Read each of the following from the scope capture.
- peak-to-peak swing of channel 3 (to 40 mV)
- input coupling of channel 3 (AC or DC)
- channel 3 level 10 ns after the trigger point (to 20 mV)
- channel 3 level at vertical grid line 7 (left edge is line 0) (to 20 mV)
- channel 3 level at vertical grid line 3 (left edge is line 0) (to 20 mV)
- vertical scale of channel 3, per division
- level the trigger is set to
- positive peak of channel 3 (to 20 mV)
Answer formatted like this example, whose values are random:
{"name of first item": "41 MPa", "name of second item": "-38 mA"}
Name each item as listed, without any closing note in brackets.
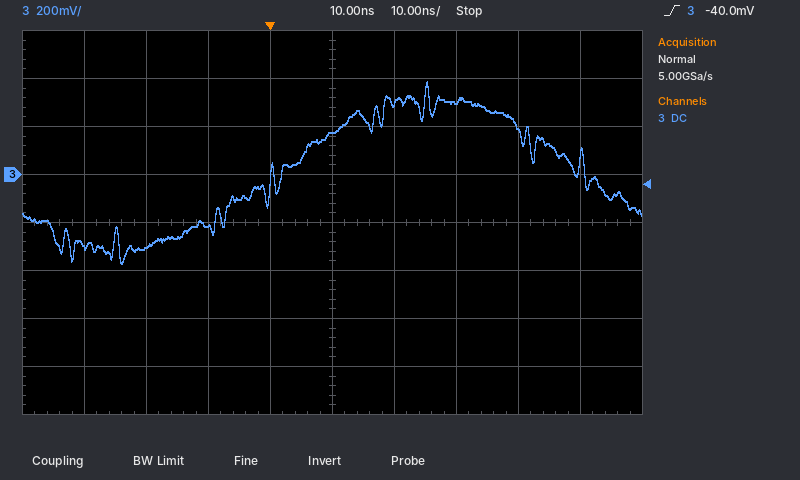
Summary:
{"peak-to-peak swing of channel 3": "760 mV", "input coupling of channel 3": "DC", "channel 3 level 10 ns after the trigger point": "180 mV", "channel 3 level at vertical grid line 7 (left edge is line 0)": "300 mV", "channel 3 level at vertical grid line 3 (left edge is line 0)": "-220 mV", "vertical scale of channel 3, per division": "200 mV", "level the trigger is set to": "-40.0 mV", "positive peak of channel 3": "380 mV"}
